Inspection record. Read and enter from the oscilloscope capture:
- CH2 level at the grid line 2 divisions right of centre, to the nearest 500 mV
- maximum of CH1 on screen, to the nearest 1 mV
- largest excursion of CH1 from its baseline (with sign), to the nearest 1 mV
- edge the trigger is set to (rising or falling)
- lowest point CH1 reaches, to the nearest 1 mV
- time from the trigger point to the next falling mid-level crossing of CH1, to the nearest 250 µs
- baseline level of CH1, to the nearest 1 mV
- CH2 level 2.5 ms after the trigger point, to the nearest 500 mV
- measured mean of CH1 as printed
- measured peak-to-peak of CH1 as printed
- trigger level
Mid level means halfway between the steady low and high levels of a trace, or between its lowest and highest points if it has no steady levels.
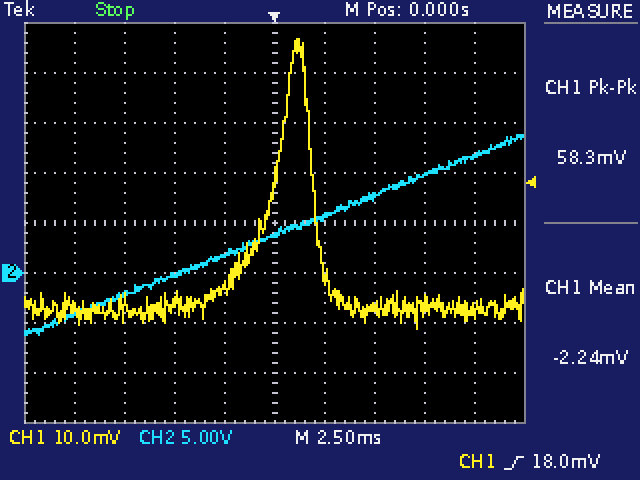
7.5 V
47 mV
+54 mV
rising
-11 mV
2.00 ms
-7 mV
5.5 V
-2.24 mV
58.3 mV
18.0 mV
